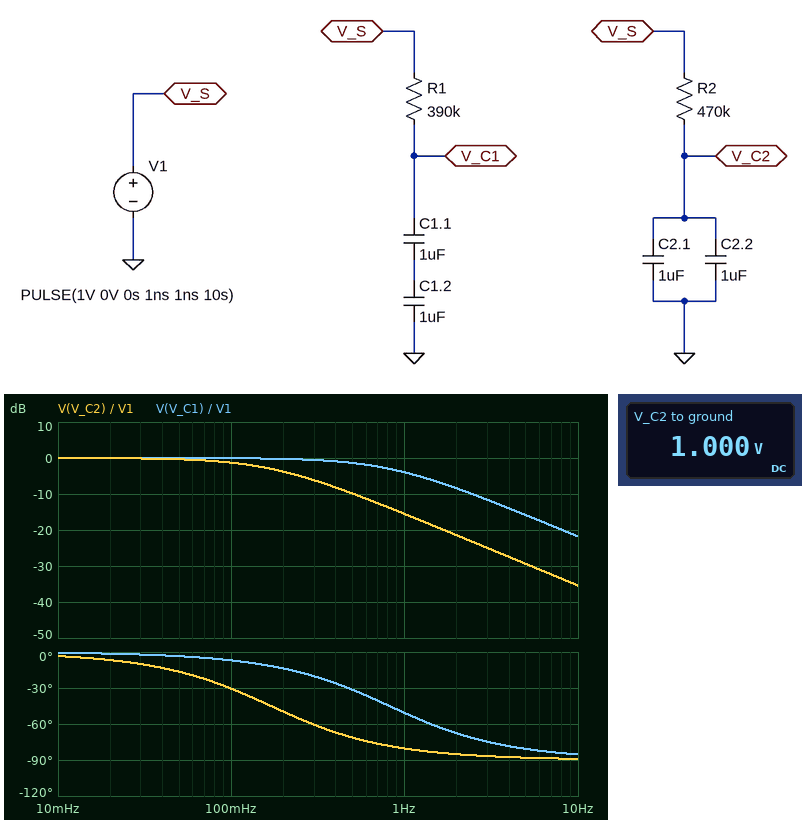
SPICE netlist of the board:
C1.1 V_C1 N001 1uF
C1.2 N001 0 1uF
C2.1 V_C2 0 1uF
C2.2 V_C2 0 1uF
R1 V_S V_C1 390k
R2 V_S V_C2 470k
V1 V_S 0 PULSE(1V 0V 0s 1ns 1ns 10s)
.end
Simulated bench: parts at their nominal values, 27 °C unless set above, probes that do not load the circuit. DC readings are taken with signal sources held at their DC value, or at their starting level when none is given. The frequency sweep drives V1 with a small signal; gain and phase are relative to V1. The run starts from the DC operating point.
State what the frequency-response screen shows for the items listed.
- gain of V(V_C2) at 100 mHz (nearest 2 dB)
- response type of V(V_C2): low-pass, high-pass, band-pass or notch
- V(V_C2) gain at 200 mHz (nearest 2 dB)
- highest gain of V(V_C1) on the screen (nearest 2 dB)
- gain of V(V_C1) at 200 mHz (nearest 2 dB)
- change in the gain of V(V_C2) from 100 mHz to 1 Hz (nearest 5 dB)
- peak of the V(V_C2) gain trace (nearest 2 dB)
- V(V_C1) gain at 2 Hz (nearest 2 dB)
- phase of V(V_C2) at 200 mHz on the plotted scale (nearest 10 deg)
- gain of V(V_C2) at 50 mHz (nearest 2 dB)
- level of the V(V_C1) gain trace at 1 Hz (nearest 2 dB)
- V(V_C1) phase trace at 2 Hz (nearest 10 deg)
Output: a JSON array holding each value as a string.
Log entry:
["-2 dB", "low-pass", "-4 dB", "0 dB", "0 dB", "-15 dB", "0 dB", "-8 dB", "-50 deg", "0 dB", "-4 dB", "-70 deg"]
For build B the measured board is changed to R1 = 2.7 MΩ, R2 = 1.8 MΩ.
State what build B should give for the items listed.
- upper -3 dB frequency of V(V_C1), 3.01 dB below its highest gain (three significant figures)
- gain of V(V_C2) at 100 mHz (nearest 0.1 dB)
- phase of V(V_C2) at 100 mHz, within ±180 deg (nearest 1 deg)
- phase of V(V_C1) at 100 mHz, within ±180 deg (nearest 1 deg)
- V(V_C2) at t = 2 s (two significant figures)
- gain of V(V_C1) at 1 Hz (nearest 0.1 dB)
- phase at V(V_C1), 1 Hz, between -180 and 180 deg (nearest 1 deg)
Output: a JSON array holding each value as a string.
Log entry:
["118 mHz", "-7.9 dB", "-66 deg", "-40 deg", "570 mV", "-18.6 dB", "-83 deg"]
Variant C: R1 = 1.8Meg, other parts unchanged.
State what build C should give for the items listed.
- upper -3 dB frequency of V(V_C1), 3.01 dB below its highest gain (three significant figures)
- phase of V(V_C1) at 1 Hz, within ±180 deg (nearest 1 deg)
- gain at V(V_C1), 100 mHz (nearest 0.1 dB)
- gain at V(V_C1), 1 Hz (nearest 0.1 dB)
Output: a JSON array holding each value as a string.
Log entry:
["177 mHz", "-80 deg", "-1.2 dB", "-15.2 dB"]
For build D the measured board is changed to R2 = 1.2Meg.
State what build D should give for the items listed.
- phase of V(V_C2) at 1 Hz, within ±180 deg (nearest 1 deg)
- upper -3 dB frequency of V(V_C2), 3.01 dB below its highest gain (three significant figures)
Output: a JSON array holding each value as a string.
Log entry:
["-86 deg", "66.3 mHz"]
